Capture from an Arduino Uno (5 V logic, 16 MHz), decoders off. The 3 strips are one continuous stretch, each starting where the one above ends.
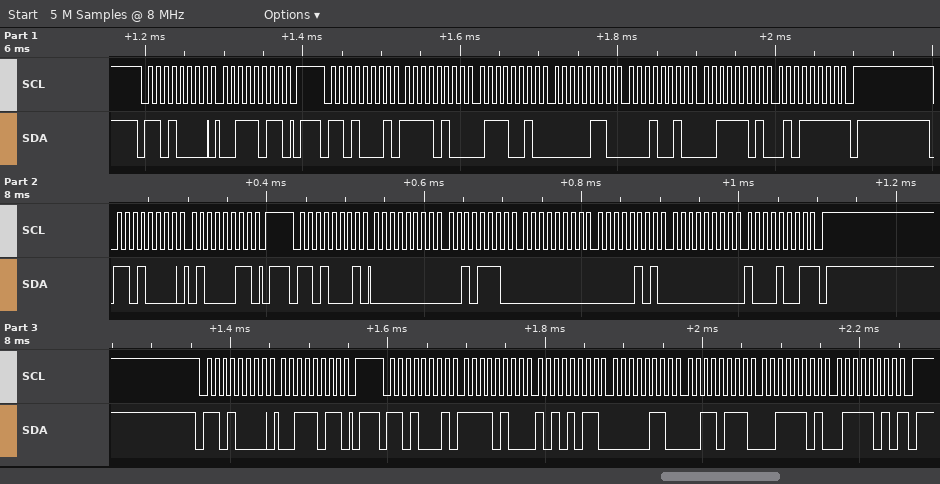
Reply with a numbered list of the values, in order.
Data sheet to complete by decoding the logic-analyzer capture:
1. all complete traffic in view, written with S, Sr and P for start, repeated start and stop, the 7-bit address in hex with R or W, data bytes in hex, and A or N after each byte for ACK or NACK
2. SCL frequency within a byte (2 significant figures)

1. S 68W A 3B A P S 68R A F4 A 72 A 06 A 12 A 3D A 5F N P S 68W A 43 A P S 68R A 00 A 2E A 00 A 05 A 00 A 89 N P S 68W A 3B A P S 68R A F4 A AB A 06 A 37 A 3D A 7A N P
2. 100 kHz
